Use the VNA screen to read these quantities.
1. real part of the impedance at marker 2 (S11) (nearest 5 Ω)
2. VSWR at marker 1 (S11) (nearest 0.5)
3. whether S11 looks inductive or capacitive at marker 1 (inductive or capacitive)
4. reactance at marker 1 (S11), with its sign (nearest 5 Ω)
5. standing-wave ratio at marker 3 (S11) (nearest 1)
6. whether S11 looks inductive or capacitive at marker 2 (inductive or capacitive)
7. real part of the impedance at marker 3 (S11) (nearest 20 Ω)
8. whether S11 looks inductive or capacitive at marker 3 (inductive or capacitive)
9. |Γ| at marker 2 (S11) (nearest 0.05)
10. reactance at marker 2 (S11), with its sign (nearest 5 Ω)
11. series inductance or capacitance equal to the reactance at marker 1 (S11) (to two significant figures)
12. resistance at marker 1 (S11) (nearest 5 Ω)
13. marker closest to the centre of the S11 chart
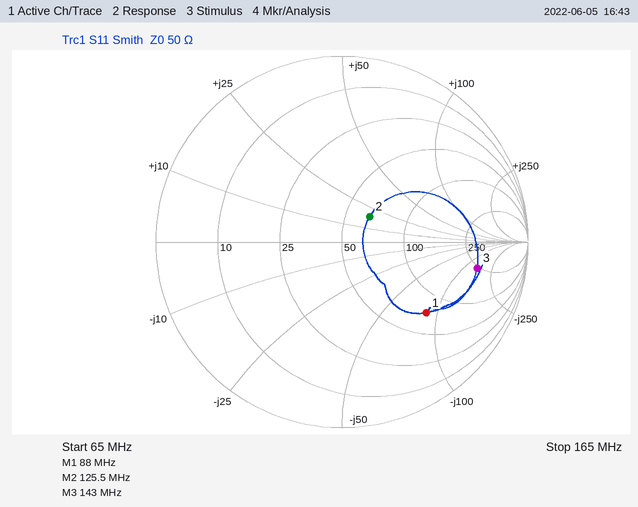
65 Ω
4.0
capacitive
-85 Ω
7
inductive
240 Ω
capacitive
0.20
+20 Ω
21 pF
75 Ω
marker 2
